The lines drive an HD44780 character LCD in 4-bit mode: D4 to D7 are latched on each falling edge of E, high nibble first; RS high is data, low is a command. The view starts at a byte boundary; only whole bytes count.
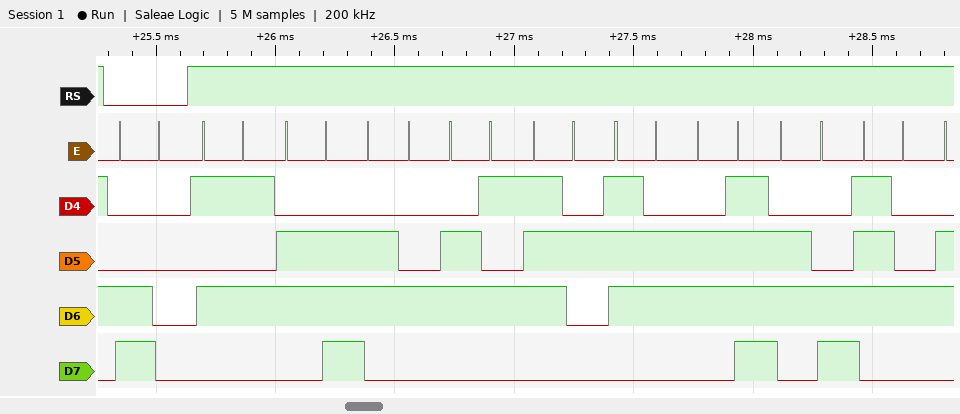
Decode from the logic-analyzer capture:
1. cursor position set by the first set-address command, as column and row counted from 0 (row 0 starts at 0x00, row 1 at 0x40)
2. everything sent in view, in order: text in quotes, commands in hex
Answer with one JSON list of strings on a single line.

["column 0, row 1", "0xC0 \"Undervolt\""]
